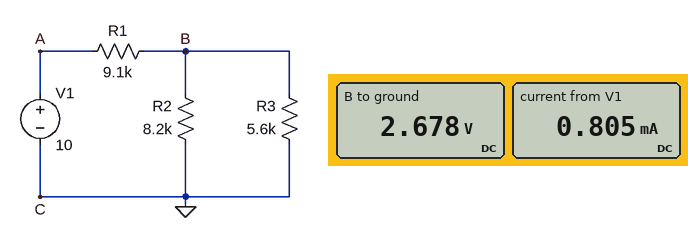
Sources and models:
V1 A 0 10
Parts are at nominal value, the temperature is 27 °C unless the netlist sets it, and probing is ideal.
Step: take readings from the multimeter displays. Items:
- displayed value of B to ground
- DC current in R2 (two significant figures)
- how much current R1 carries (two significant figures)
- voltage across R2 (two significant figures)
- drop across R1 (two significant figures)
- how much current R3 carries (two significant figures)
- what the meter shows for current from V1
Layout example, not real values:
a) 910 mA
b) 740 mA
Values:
a) 2.678 V
b) 330 µA
c) 800 µA
d) 2.7 V
e) 7.3 V
f) 480 µA
g) 0.805 mA
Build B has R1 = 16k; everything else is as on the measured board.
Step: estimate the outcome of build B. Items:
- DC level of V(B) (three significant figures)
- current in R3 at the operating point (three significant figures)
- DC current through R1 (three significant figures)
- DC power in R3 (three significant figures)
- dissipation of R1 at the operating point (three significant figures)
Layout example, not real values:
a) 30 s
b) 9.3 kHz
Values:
a) 1.72 V
b) 307 µA
c) 517 µA
d) 529 µW
e) 4.28 mW
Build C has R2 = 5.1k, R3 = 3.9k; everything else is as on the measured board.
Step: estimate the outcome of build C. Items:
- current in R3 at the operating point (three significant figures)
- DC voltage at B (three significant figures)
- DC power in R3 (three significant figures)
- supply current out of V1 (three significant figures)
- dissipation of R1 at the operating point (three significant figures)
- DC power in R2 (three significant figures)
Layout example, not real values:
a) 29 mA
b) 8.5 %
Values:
a) 501 µA
b) 1.95 V
c) 979 µW
d) 884 µA
e) 7.11 mW
f) 749 µW
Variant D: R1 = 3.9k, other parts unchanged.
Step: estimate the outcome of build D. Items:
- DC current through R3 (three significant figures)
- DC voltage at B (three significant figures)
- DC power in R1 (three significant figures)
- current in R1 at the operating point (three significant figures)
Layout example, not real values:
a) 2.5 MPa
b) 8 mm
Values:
a) 822 µA
b) 4.60 V
c) 7.47 mW
d) 1.38 mA
